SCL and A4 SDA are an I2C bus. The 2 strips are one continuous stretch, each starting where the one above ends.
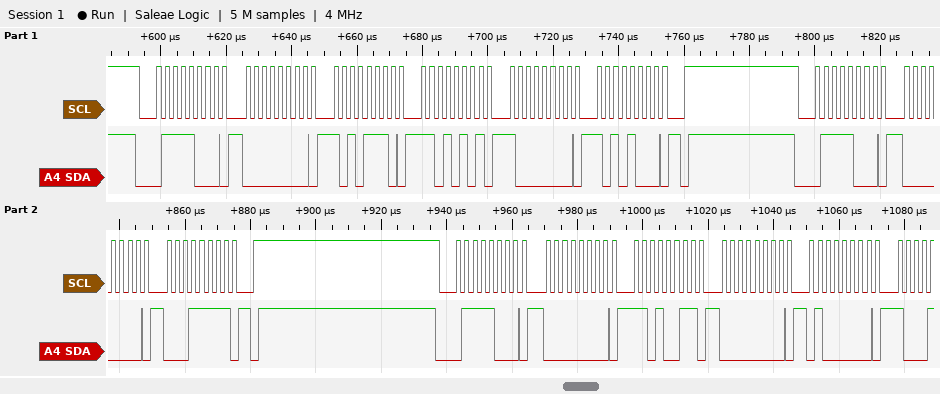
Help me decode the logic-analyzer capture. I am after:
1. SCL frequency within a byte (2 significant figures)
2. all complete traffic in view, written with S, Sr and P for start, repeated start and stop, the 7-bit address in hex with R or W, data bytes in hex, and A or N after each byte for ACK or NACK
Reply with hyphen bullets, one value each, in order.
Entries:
- 400 kHz
- S 3CW A 00 A AE A D5 A 80 A A8 A P S 3CW A 00 A 1F A P S 3CW A 00 A D3 A 00 A 40 A
